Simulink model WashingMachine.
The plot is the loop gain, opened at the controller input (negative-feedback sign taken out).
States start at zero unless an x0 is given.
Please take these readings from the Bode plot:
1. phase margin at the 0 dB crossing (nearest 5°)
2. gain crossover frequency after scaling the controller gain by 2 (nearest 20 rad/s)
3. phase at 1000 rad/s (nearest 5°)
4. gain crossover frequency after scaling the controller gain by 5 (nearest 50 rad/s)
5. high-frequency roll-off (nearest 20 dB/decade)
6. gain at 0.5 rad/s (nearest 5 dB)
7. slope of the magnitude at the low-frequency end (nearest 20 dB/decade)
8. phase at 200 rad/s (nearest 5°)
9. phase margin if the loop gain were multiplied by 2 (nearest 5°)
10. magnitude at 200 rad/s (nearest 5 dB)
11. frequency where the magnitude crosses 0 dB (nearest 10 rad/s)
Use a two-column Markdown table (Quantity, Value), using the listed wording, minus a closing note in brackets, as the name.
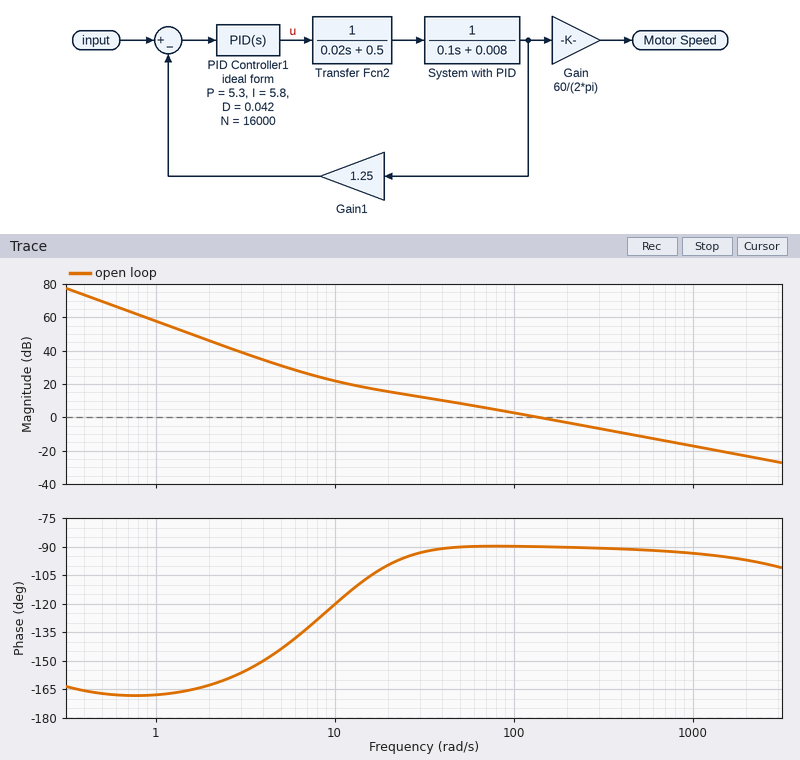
| Quantity | Value |
|---|---|
| phase margin at the 0 dB crossing | 90° |
| gain crossover frequency after scaling the controller gain by 2 | 280 rad/s |
| phase at 1000 rad/s | -95° |
| gain crossover frequency after scaling the controller gain by 5 | 700 rad/s |
| high-frequency roll-off | -20 dB/decade |
| gain at 0.5 rad/s | 70 dB |
| slope of the magnitude at the low-frequency end | -40 dB/decade |
| phase at 200 rad/s | -90° |
| phase margin if the loop gain were multiplied by 2 | 90° |
| magnitude at 200 rad/s | -5 dB |
| frequency where the magnitude crosses 0 dB | 140 rad/s |
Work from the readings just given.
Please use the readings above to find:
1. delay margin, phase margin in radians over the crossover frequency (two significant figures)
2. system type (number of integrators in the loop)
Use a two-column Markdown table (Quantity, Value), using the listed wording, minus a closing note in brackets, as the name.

| Quantity | Value |
|---|---|
| delay margin, phase margin in radians over the crossover frequency | 0.011 s |
| system type | 2 |
